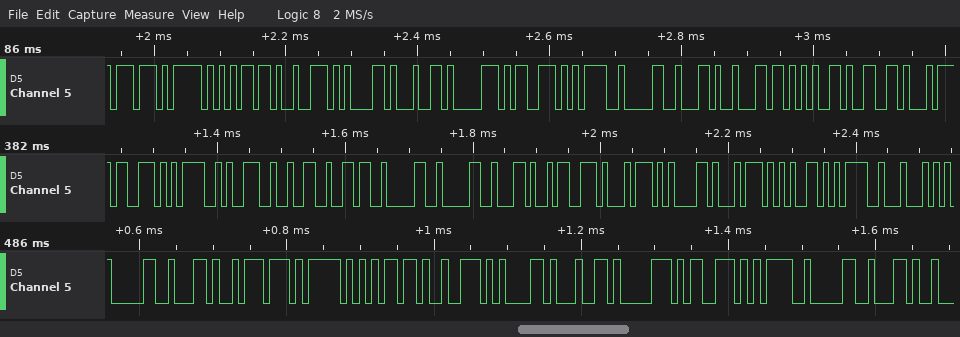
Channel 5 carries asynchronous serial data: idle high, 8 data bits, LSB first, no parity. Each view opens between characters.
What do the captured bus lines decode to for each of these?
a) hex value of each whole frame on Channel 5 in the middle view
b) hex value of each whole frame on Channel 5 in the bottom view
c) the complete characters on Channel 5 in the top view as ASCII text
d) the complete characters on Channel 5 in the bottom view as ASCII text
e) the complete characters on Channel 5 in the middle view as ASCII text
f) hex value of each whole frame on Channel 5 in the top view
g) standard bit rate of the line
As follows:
73, 3D, 39, 32, 36, 30, 30, 2C, 73, 74, 61, 74, 65, 3D, 44
30, 2C, 77, 5F, 6D, 72, 61, 64, 70, 73, 3D, 30, 2C
"w_mradps=0,lef"
"0,w_mradps=0,"
"s=92600,state=D"
77, 5F, 6D, 72, 61, 64, 70, 73, 3D, 30, 2C, 6C, 65, 66
115200 baud
